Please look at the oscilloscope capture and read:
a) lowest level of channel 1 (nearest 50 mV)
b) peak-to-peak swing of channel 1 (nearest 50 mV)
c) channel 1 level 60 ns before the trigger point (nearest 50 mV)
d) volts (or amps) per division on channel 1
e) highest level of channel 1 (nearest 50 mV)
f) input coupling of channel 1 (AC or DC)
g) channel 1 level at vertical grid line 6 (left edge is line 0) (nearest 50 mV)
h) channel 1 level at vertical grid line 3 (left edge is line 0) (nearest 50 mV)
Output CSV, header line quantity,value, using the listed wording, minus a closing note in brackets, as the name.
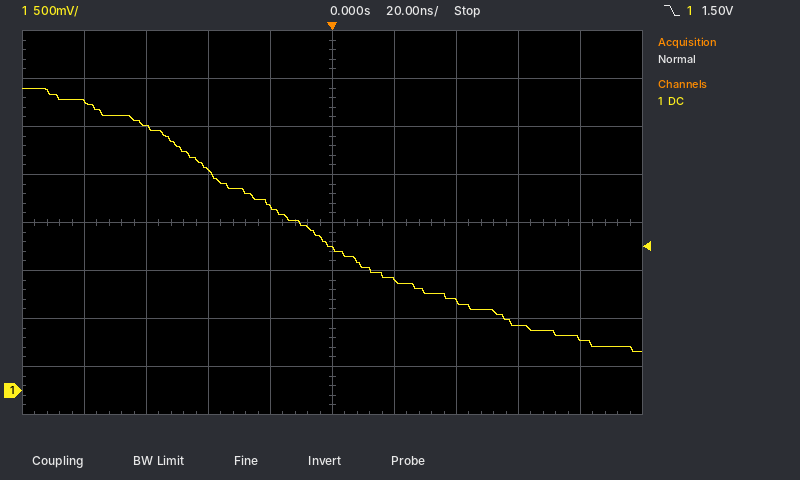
quantity,value
lowest level of channel 1,400 mV
peak-to-peak swing of channel 1,2.75 V
channel 1 level 60 ns before the trigger point,2.75 V
volts (or amps) per division on channel 1,500 mV
highest level of channel 1,3.15 V
input coupling of channel 1,DC
channel 1 level at vertical grid line 6 (left edge is line 0),1.15 V
channel 1 level at vertical grid line 3 (left edge is line 0),2.30 V
